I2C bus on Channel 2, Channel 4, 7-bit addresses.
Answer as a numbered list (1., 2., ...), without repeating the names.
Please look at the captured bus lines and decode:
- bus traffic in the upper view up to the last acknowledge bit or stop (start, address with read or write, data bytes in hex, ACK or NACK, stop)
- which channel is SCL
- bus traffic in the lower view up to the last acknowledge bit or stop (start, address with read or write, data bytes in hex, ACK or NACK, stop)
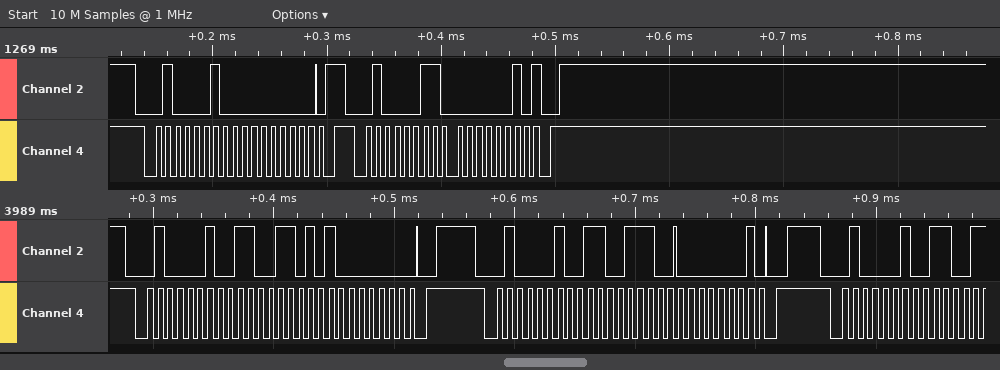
1. start, address 21 write ACK, 00 ACK, repeated start, address 21 read ACK, 02 NACK, stop
2. Channel 4
3. start, address 21 write ACK, CD ACK, 80 ACK, stop, start, address 21 write ACK, CE ACK, 01 ACK, stop, start, address 21 write ACK
